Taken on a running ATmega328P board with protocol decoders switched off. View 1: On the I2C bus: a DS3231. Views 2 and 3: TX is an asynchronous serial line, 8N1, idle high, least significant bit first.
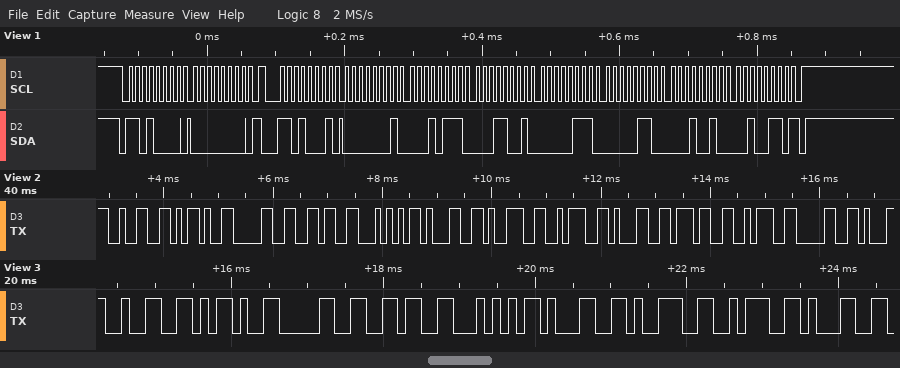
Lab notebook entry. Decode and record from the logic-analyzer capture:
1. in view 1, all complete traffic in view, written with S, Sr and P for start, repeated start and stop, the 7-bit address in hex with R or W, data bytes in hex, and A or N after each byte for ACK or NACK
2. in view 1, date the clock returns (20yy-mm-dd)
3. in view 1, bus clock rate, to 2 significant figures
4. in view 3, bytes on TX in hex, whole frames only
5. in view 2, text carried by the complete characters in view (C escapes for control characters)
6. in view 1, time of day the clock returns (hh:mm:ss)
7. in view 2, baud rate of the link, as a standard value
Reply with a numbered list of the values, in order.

1. S 68W A 00 A Sr 68R A 01 A 17 A 19 A 07 A 06 A 12 A 26 N P
2. 2026-12-06
3. 100 kHz
4. 0x32 0x2D 0x30 0x36 0x54 0x31 0x39 0x3A 0x31
5. "2-06T19:17:0"
6. 19:17:01
7. 9600 baud
